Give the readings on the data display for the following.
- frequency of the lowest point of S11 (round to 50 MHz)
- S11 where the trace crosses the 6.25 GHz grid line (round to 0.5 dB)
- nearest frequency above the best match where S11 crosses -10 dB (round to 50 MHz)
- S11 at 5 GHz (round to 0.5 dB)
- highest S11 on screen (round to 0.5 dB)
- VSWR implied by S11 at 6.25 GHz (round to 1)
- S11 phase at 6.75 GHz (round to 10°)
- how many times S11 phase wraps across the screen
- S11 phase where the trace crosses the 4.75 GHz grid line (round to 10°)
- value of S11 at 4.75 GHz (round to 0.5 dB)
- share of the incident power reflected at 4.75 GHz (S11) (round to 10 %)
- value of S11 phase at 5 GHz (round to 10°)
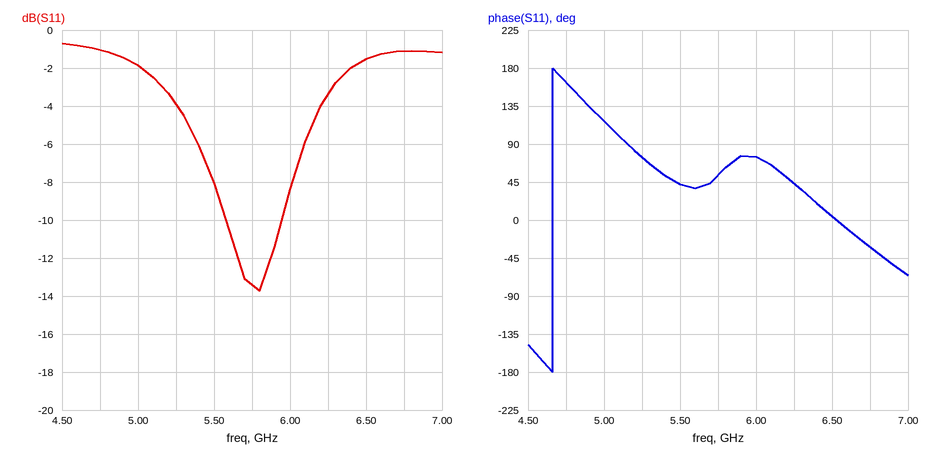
5.80 GHz
-3.5 dB
5.95 GHz
-2.0 dB
-0.5 dB
5
-30°
1
160°
-1.0 dB
80 %
120°
